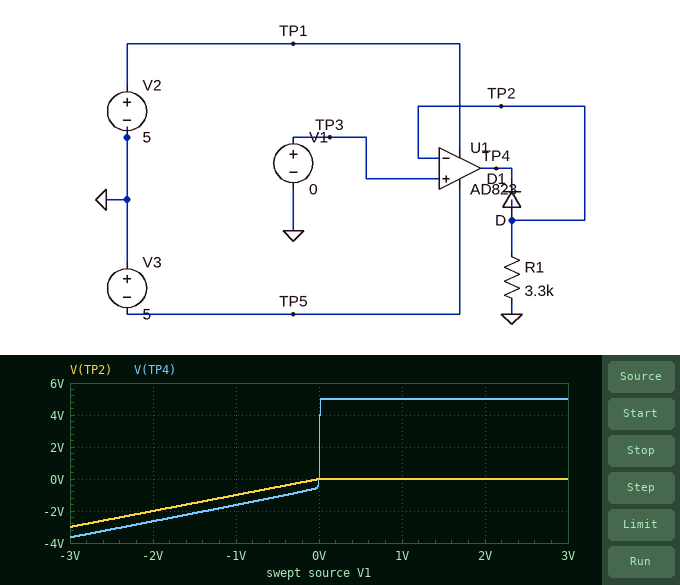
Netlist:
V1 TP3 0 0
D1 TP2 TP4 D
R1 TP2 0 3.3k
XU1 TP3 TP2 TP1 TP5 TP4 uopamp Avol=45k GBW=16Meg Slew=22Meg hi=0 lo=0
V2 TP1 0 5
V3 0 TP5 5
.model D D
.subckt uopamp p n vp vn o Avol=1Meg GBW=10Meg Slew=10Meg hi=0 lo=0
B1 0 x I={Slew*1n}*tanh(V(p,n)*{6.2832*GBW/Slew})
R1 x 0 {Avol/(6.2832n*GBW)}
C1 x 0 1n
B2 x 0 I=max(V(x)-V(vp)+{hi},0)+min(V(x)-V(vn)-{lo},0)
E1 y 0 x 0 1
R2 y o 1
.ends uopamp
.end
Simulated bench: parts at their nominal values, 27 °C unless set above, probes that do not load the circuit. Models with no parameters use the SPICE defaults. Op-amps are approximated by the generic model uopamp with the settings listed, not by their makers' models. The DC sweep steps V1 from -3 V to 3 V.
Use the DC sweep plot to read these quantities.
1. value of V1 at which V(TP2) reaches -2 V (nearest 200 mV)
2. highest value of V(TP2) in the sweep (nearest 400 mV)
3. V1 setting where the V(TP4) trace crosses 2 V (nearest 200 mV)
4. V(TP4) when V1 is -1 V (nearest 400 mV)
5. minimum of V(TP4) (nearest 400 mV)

-2.0 V
0 V
0 V
-1.6 V
-3.6 V
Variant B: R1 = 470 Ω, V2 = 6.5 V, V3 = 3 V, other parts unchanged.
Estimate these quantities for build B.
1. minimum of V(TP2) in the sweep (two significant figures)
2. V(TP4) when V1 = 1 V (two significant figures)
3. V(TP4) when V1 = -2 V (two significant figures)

-2.3 V
6.5 V
-2.7 V
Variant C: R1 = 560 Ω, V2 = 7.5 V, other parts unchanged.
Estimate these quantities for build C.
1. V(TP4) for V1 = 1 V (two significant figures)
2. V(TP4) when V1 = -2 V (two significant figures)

7.5 V
-2.7 V
